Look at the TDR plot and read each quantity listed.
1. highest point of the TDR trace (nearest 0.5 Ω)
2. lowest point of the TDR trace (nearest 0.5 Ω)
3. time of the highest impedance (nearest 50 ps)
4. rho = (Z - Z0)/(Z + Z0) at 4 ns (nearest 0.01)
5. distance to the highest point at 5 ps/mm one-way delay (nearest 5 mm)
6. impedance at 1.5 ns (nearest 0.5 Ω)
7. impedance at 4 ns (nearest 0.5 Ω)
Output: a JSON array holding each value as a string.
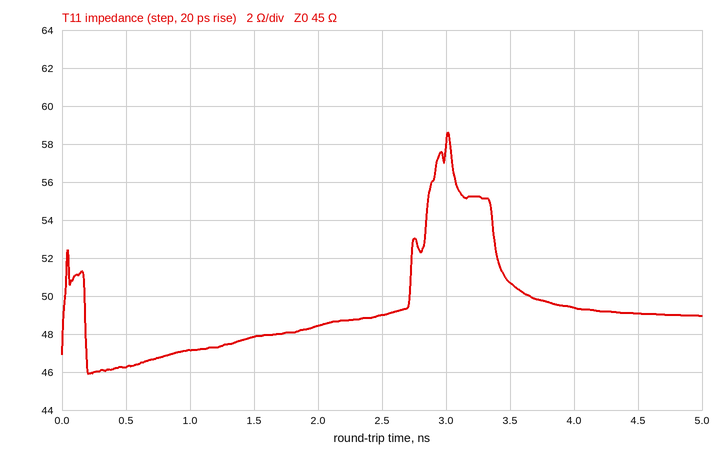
["58.5 Ω", "46.0 Ω", "3.00 ns", "+0.05", "300 mm", "48.0 Ω", "49.5 Ω"]
